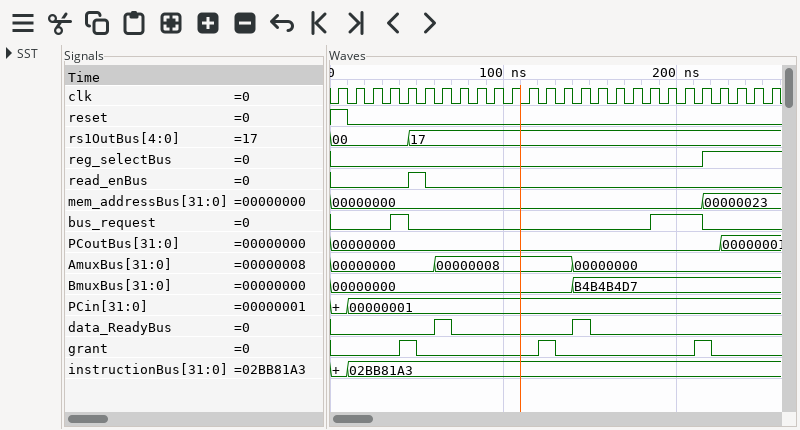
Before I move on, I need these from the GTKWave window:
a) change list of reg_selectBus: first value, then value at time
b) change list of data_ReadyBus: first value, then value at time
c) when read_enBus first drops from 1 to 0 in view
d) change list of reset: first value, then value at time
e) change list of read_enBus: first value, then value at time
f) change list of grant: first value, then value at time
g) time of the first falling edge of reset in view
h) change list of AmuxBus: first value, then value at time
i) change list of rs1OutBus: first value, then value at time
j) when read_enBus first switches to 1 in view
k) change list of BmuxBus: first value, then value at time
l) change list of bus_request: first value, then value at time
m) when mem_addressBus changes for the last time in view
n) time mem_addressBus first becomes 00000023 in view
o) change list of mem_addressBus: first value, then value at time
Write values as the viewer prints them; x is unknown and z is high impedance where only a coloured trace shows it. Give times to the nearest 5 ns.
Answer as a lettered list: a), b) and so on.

a) 0, 1 at 215 ns
b) 0, 1 at 60 ns, 0 at 70 ns, 1 at 140 ns, 0 at 150 ns
c) 55 ns
d) 1, 0 at 10 ns
e) 0, 1 at 45 ns, 0 at 55 ns
f) 0, 1 at 40 ns, 0 at 50 ns, 1 at 120 ns, 0 at 130 ns, 1 at 210 ns, 0 at 220 ns
g) 10 ns
h) 00000000, 00000008 at 60 ns, 00000000 at 140 ns
i) 00, 17 at 45 ns
j) 45 ns
k) 00000000, B4B4B4D7 at 140 ns
l) 0, 1 at 35 ns, 0 at 45 ns, 1 at 185 ns, 0 at 215 ns
m) 215 ns
n) 215 ns
o) 00000000, 00000023 at 215 ns
